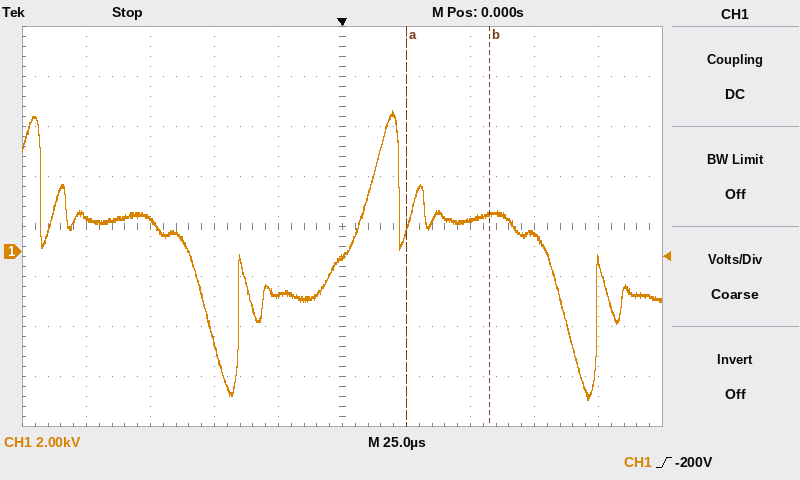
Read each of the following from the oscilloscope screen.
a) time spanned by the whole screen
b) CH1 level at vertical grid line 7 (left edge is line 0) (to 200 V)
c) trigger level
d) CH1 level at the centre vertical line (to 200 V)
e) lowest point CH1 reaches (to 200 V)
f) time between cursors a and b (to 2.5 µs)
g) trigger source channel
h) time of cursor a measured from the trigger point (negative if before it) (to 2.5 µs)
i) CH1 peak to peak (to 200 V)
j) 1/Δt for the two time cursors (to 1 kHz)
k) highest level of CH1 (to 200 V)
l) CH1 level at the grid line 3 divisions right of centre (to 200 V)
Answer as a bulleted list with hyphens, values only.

- 250 µs
- 1.2 kV
- -200 V
- -200 V
- -6.0 kV
- 32.5 µs
- CH1
- +25.0 µs
- 11.6 kV
- 31 kHz
- 5.6 kV
- 800 V
